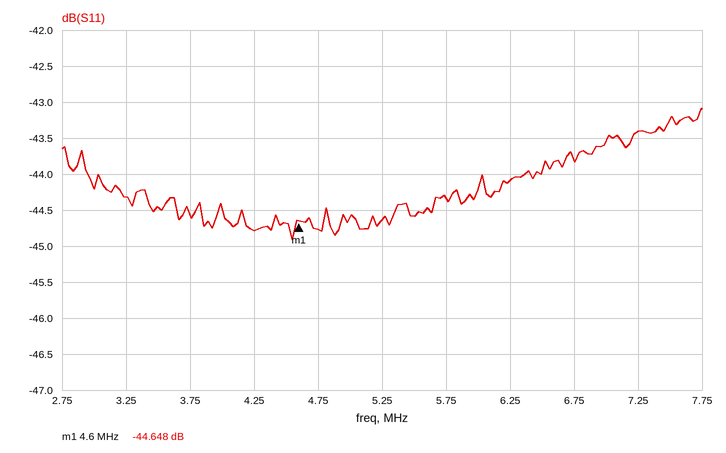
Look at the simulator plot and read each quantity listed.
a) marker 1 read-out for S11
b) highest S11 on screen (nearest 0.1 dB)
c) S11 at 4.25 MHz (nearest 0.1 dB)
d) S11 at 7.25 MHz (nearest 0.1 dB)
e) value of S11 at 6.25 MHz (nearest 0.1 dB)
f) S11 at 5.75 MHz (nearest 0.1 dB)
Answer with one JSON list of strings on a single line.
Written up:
["-44.648 dB", "-43.1 dB", "-44.8 dB", "-43.4 dB", "-44.1 dB", "-44.3 dB"]
